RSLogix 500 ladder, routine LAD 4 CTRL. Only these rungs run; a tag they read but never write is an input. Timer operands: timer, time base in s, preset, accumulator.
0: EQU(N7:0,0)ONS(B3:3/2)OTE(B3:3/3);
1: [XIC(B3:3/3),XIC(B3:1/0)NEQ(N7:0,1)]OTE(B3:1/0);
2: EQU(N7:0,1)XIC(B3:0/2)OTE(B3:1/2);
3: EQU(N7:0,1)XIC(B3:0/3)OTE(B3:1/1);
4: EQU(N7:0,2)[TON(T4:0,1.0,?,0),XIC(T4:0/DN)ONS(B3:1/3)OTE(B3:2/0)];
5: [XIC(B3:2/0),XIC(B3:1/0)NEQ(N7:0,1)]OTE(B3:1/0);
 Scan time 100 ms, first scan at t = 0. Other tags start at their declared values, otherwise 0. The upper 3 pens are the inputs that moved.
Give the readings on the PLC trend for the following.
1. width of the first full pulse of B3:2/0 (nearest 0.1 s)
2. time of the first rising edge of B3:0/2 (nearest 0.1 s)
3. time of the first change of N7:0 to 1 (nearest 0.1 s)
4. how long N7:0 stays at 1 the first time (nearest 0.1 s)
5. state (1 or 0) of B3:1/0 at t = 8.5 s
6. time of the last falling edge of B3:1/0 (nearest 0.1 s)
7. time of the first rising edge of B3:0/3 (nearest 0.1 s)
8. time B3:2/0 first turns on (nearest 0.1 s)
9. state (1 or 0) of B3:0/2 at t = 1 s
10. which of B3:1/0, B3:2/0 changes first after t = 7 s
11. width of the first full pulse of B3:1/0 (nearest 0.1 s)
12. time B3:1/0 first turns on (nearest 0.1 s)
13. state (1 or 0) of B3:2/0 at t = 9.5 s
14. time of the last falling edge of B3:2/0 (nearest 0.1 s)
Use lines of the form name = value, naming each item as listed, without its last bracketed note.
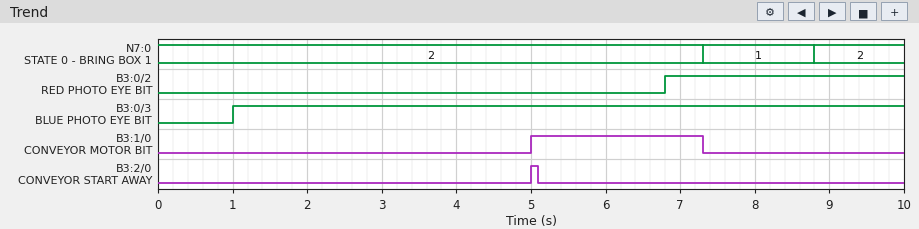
width of the first full pulse of B3:2/0 = 0.1 s
time of the first rising edge of B3:0/2 = 6.8 s
time of the first change of N7:0 to 1 = 7.3 s
how long N7:0 stays at 1 the first time = 1.5 s
state (1 or 0) of B3:1/0 at t = 8.5 s = 0
time of the last falling edge of B3:1/0 = 7.3 s
time of the first rising edge of B3:0/3 = 1.0 s
time B3:2/0 first turns on = 5.0 s
state (1 or 0) of B3:0/2 at t = 1 s = 0
which of B3:1/0, B3:2/0 changes first after t = 7 s = B3:1/0
width of the first full pulse of B3:1/0 = 2.3 s
time B3:1/0 first turns on = 5.0 s
state (1 or 0) of B3:2/0 at t = 9.5 s = 0
time of the last falling edge of B3:2/0 = 5.1 s
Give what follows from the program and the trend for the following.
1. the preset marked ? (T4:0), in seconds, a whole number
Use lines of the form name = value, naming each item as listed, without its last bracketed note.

the preset marked ? (T4:0), in seconds, a whole number = 5 s
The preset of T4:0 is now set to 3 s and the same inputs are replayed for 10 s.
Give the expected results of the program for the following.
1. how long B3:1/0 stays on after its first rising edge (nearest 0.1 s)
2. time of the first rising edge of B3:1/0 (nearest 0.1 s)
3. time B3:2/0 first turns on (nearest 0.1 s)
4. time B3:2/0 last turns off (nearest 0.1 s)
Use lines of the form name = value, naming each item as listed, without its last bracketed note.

how long B3:1/0 stays on after its first rising edge = 4.3 s
time of the first rising edge of B3:1/0 = 3.0 s
time B3:2/0 first turns on = 3.0 s
time B3:2/0 last turns off = 3.1 s
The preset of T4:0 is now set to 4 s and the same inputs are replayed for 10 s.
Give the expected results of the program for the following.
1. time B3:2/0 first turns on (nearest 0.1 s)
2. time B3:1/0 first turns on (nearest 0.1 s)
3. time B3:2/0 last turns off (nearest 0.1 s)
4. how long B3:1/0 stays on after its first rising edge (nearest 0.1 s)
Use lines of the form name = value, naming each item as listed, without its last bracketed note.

time B3:2/0 first turns on = 4.0 s
time B3:1/0 first turns on = 4.0 s
time B3:2/0 last turns off = 4.1 s
how long B3:1/0 stays on after its first rising edge = 3.3 s
